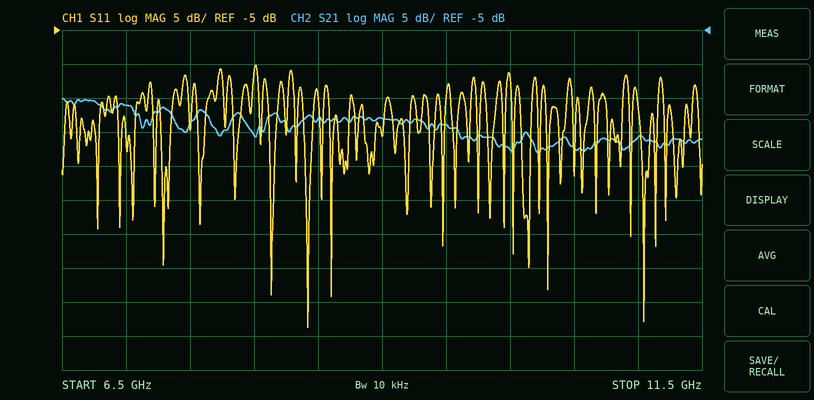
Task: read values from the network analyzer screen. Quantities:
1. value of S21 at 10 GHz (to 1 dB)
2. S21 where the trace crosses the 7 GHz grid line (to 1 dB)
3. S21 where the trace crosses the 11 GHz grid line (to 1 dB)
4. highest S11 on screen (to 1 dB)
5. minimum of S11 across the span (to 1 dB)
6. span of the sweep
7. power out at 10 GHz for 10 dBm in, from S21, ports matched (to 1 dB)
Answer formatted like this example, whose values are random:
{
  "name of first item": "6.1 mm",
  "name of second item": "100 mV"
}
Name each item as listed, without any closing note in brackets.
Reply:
{
  "value of S21 at 10 GHz": "-23 dB",
  "S21 where the trace crosses the 7 GHz grid line": "-16 dB",
  "S21 where the trace crosses the 11 GHz grid line": "-21 dB",
  "highest S11 on screen": "-10 dB",
  "minimum of S11 across the span": "-49 dB",
  "span of the sweep": "5 GHz",
  "power out at 10 GHz for 10 dBm in, from S21, ports matched": "-13 dBm"
}
